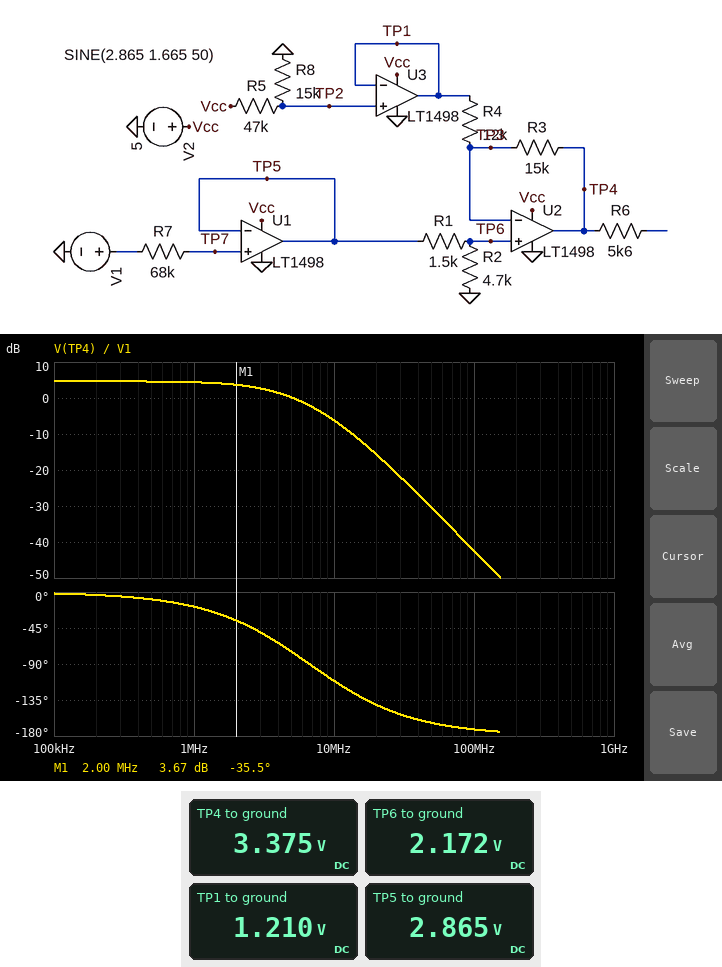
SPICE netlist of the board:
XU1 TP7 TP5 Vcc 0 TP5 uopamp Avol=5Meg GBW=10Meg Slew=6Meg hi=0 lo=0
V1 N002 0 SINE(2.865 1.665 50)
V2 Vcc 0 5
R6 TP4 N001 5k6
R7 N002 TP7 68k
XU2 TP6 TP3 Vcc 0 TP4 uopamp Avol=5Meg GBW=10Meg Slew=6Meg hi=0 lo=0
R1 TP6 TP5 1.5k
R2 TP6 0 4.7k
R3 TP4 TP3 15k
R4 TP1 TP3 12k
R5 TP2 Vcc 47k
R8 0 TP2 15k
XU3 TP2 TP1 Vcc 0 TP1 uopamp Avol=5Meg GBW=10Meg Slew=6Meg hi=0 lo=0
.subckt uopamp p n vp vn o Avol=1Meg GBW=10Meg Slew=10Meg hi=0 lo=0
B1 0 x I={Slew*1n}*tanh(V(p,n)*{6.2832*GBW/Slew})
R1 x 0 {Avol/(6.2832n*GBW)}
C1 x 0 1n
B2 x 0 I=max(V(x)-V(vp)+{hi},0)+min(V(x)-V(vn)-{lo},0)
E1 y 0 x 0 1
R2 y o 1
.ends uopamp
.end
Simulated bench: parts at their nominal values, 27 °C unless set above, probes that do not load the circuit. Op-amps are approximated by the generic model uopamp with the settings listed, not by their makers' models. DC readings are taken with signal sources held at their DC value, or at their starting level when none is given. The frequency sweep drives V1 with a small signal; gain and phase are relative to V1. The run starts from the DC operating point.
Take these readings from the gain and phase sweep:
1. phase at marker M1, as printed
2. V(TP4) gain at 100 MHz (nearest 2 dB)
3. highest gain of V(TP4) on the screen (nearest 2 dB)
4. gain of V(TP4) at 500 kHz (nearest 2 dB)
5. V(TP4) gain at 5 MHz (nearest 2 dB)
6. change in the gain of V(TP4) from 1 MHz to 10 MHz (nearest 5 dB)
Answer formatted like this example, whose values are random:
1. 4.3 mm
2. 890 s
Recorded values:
1. -35.5 deg
2. -42 dB
3. 4 dB
4. 4 dB
5. 0 dB
6. -10 dB
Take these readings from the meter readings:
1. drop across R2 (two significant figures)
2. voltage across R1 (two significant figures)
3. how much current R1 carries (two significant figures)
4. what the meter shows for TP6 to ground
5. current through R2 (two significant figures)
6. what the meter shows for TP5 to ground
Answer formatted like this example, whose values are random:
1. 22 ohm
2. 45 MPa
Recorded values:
1. 2.2 V
2. 690 mV
3. 460 µA
4. 2.172 V
5. 460 µA
6. 2.865 V
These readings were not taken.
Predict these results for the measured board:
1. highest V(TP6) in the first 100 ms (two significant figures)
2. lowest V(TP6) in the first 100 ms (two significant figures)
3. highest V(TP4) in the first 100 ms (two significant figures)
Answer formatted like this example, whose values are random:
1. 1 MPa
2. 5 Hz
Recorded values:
1. 3.4 V
2. 910 mV
3. 5.0 V
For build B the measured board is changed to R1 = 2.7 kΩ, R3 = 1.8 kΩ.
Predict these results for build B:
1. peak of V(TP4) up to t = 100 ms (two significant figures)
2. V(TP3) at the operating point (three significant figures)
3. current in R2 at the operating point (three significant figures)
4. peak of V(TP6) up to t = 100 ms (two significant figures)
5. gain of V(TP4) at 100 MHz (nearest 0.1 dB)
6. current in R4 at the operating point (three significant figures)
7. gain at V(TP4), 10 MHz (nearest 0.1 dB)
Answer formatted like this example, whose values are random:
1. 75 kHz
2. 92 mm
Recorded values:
1. 3.1 V
2. 1.82 V
3. 387 µA
4. 2.9 V
5. -44.0 dB
6. 50.8 µA
7. -9.4 dB
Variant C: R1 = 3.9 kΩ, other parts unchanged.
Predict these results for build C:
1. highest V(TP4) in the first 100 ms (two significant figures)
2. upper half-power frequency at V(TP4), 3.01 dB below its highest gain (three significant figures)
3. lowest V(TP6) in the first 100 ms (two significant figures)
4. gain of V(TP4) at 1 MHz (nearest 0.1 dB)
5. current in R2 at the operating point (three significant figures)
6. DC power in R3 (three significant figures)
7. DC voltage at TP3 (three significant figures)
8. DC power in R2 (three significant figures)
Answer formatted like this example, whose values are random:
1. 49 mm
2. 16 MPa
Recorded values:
1. 4.1 V
2. 3.83 MHz
3. 660 mV
4. 1.5 dB
5. 333 µA
6. 13.2 µW
7. 1.57 V
8. 522 µW
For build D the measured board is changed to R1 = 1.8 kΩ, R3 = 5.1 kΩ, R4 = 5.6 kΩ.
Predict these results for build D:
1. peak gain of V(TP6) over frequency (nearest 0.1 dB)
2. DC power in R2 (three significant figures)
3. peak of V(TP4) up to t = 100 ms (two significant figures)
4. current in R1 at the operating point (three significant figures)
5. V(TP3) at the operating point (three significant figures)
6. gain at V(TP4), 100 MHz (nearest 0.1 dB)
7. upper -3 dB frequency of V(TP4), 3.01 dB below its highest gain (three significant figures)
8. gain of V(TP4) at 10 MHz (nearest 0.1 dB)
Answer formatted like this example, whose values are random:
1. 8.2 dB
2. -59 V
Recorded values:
1. -2.8 dB
2. 913 µW
3. 5.0 V
4. 441 µA
5. 2.07 V
6. -42.9 dB
7. 4.33 MHz
8. -6.9 dB
